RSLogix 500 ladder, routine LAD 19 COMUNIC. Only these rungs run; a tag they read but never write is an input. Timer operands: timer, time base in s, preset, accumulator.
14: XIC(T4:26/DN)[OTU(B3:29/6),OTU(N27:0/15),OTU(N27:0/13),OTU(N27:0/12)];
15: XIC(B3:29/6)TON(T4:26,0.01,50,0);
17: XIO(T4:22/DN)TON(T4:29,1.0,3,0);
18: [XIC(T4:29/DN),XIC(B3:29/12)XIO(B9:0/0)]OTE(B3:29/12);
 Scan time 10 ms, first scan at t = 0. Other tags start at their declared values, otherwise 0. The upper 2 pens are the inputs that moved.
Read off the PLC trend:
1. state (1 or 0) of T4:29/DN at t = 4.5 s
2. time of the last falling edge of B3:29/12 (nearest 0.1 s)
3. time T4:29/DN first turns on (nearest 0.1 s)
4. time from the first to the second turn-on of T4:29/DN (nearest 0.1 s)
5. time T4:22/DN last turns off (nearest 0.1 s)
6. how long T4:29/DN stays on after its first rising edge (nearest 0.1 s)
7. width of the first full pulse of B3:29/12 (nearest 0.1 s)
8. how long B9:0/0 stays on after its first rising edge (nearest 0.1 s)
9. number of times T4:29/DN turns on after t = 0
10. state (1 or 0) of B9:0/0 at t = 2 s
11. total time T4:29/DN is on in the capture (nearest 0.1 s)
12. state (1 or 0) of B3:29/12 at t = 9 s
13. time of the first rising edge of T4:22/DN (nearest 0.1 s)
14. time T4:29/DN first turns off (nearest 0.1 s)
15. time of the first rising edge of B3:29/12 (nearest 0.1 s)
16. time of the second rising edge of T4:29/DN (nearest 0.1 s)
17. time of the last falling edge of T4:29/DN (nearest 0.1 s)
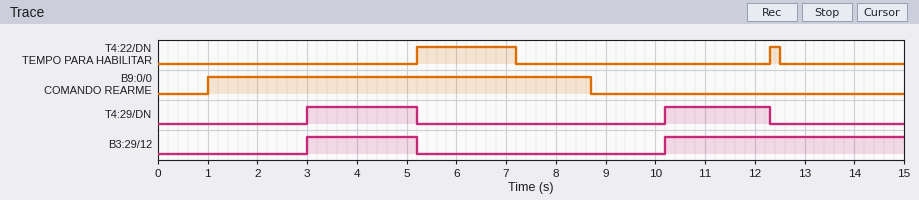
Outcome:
1
5.2 s
3.0 s
7.2 s
12.5 s
2.2 s
2.2 s
7.7 s
2
1
4.3 s
0
5.2 s
5.2 s
3.0 s
10.2 s
12.3 s
